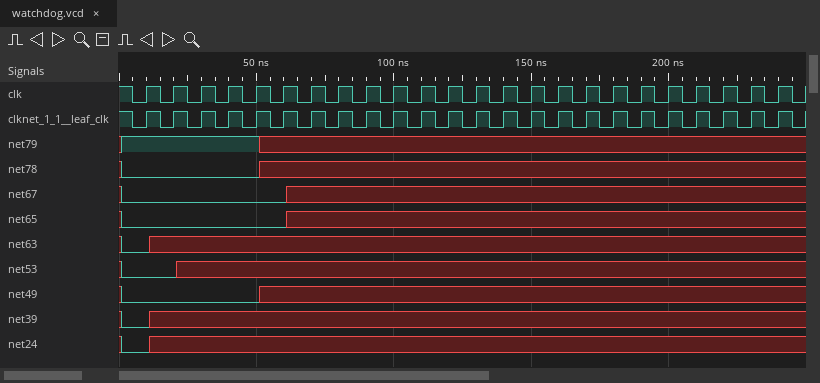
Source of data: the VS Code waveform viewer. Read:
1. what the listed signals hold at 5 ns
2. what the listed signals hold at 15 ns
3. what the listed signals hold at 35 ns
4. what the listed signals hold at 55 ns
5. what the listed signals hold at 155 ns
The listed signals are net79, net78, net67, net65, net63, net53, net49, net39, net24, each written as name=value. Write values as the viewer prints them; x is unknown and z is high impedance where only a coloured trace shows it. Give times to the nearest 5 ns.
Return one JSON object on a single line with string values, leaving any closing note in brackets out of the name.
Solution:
{"what the listed signals hold at 5 ns": "net79=1, net78=0, net67=0, net65=0, net63=0, net53=0, net49=0, net39=0, net24=0", "what the listed signals hold at 15 ns": "net79=1, net78=0, net67=0, net65=0, net63=x, net53=0, net49=0, net39=x, net24=x", "what the listed signals hold at 35 ns": "net79=1, net78=0, net67=0, net65=0, net63=x, net53=x, net49=0, net39=x, net24=x", "what the listed signals hold at 55 ns": "net79=x, net78=x, net67=0, net65=0, net63=x, net53=x, net49=x, net39=x, net24=x", "what the listed signals hold at 155 ns": "net79=x, net78=x, net67=x, net65=x, net63=x, net53=x, net49=x, net39=x, net24=x"}
